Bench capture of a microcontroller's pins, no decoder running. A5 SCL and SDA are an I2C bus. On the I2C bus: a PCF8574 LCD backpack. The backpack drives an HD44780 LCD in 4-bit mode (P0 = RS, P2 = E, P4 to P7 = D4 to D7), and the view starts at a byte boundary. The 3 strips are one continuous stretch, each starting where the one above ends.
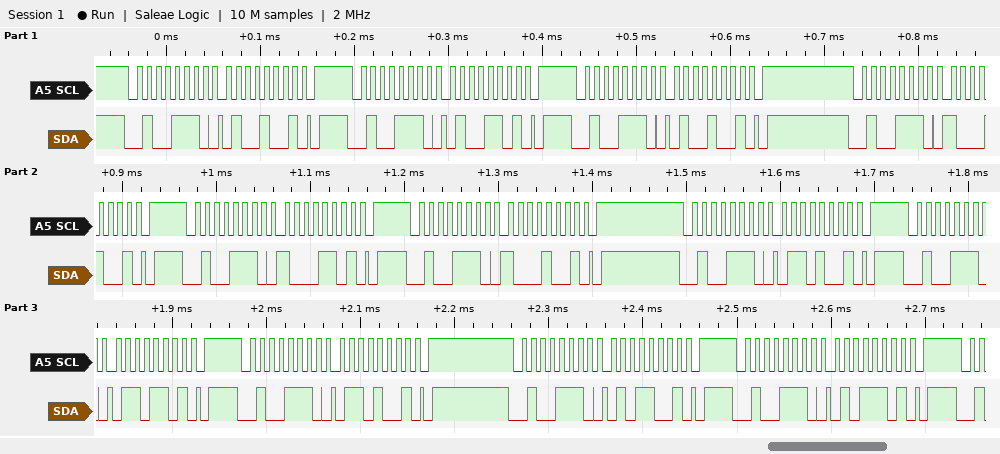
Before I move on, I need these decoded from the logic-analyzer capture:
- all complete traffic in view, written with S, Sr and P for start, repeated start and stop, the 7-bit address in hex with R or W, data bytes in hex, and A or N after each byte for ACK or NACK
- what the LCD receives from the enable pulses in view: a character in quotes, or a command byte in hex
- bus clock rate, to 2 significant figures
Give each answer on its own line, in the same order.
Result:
S 27W A 49 A P S 27W A 4D A P S 27W A 49 A P S 27W A 89 A P S 27W A 8D A P S 27W A 89 A P S 27W A 69 A P S 27W A 6D A P S 27W A 69 A P S 27W A 59 A P S 27W A 5D A P
'H'
100 kHz
